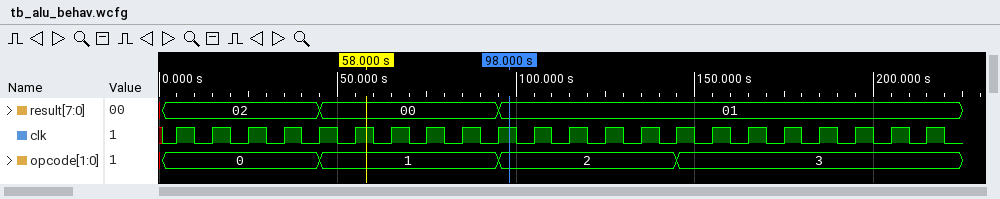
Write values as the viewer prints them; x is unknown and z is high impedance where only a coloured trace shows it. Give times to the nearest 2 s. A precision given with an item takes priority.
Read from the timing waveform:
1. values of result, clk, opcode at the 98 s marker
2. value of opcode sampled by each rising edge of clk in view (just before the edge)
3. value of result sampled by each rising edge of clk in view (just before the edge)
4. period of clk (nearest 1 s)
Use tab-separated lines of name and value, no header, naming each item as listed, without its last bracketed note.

values of result, clk, opcode at the 98 s marker	result=01, clk=1, opcode=2
value of opcode sampled by each rising edge of clk in view	0, 0, 0, 0, 0, 1, 1, 1, 1, 1, 2, 2, 2, 2, 2, 3, 3, 3, 3, 3, 3, 3
value of result sampled by each rising edge of clk in view	02, 02, 02, 02, 02, 00, 00, 00, 00, 00, 01, 01, 01, 01, 01, 01, 01, 01, 01, 01, 01, 01
period of clk	10 s
